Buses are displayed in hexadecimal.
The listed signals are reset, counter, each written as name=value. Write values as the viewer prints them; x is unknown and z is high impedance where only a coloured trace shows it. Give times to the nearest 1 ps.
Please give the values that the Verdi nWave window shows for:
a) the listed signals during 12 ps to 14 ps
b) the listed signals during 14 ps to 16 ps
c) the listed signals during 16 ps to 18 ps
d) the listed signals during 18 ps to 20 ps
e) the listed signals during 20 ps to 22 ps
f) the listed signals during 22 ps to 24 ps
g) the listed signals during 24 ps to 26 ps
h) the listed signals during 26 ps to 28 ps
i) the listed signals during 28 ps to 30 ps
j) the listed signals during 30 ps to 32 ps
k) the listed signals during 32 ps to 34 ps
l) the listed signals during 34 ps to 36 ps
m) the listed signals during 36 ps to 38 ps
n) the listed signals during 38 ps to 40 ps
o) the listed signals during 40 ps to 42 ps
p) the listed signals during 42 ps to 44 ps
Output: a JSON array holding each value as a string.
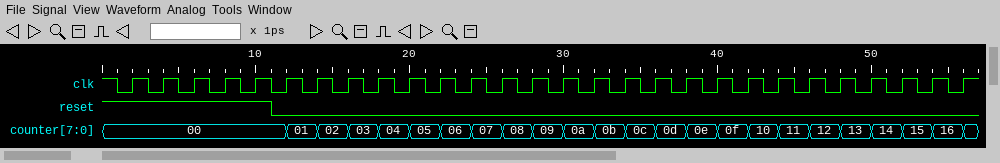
["reset=0, counter=01", "reset=0, counter=02", "reset=0, counter=03", "reset=0, counter=04", "reset=0, counter=05", "reset=0, counter=06", "reset=0, counter=07", "reset=0, counter=08", "reset=0, counter=09", "reset=0, counter=0a", "reset=0, counter=0b", "reset=0, counter=0c", "reset=0, counter=0d", "reset=0, counter=0e", "reset=0, counter=0f", "reset=0, counter=10"]
